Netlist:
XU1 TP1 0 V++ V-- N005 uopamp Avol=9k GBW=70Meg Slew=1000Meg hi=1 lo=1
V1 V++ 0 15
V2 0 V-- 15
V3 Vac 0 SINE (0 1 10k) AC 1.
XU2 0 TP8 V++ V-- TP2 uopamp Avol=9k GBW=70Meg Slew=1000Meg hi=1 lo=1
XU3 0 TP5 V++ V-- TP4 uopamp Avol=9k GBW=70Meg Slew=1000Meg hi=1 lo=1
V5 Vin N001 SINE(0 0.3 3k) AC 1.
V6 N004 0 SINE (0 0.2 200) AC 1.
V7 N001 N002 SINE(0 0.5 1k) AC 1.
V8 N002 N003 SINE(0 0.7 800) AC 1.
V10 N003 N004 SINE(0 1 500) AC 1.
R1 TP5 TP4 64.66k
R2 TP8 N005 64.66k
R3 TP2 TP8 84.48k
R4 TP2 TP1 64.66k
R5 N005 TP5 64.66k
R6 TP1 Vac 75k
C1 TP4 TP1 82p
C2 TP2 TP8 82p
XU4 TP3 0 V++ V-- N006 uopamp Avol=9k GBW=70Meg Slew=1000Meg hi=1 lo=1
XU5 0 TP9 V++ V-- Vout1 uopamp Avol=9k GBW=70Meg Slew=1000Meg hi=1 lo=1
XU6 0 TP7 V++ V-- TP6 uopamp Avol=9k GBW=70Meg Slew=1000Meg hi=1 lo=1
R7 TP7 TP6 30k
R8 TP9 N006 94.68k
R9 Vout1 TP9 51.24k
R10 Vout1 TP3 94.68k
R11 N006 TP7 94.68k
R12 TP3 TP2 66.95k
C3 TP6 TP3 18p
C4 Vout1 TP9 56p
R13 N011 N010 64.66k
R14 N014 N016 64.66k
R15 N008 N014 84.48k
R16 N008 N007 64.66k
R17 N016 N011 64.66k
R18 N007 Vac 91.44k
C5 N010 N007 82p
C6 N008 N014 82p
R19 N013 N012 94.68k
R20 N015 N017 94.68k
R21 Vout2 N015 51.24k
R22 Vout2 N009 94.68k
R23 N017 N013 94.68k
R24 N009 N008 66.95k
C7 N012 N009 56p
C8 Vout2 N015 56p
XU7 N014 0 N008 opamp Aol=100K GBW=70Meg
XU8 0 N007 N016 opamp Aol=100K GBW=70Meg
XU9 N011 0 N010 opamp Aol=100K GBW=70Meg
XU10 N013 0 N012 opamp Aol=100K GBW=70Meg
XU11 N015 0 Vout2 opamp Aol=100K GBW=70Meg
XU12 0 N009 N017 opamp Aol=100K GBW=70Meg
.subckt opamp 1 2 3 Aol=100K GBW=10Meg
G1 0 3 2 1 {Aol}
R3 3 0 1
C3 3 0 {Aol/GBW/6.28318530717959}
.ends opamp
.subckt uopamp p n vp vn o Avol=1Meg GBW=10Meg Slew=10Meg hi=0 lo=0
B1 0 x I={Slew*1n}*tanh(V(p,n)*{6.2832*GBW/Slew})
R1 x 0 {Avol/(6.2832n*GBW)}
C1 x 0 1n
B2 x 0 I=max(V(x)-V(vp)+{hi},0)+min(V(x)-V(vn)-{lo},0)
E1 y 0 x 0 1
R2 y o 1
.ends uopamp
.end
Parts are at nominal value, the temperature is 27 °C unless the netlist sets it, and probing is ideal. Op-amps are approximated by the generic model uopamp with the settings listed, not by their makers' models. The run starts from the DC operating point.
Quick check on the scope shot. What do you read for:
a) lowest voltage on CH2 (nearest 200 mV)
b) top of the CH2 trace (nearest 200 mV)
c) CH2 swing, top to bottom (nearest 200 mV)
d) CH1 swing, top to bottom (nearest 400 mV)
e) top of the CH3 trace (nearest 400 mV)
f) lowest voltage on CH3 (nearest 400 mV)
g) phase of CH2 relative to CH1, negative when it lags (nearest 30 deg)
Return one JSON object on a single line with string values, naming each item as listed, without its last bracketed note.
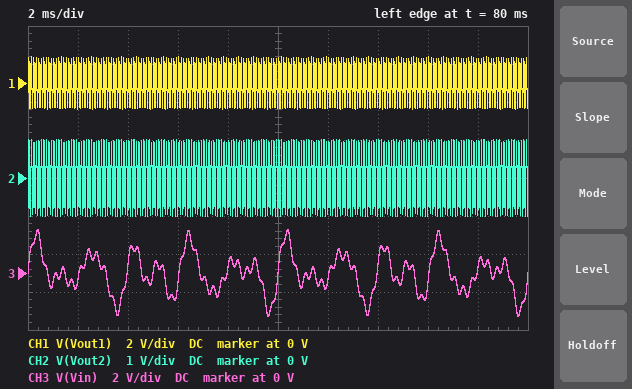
{"lowest voltage on CH2": "-1.0 V", "top of the CH2 trace": "1.0 V", "CH2 swing, top to bottom": "2.0 V", "CH1 swing, top to bottom": "2.8 V", "top of the CH3 trace": "2.4 V", "lowest voltage on CH3": "-2.4 V", "phase of CH2 relative to CH1, negative when it lags": "-30 deg"}
